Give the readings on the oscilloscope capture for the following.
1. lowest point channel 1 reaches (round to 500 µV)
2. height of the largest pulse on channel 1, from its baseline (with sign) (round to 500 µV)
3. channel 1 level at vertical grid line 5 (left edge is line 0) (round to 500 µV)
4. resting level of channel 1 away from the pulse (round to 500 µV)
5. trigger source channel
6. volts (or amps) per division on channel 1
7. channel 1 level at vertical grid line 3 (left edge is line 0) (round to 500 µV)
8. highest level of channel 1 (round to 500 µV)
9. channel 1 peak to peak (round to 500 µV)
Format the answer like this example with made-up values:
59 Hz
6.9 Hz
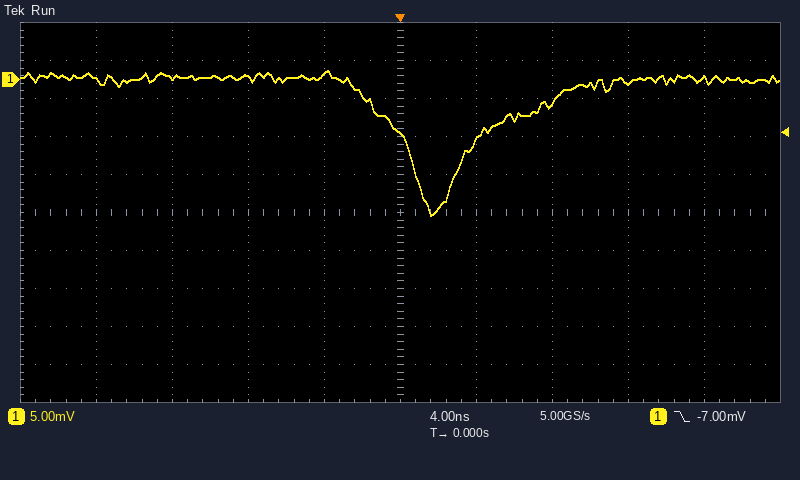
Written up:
-18.0 mV
-18.0 mV
-7.0 mV
0.0 mV
channel 1
5 mV
0.0 mV
1.0 mV
19.0 mV
